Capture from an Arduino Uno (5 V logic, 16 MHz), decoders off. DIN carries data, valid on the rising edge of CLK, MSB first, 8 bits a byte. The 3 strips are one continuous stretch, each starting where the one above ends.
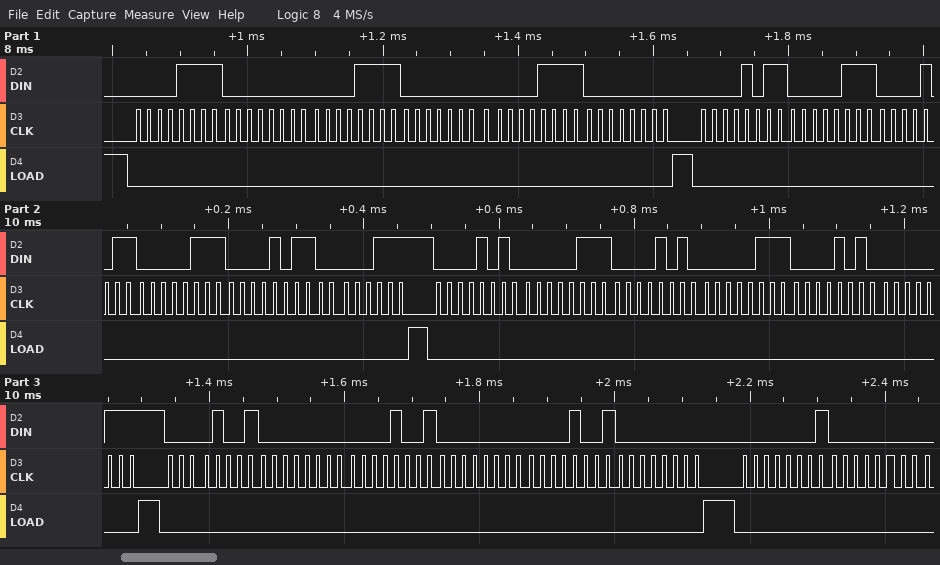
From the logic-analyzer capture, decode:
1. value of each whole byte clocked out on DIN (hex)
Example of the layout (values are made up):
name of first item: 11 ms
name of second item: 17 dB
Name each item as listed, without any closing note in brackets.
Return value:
value of each whole byte clocked out on DIN: 0x0F 0x00 0x0F 0x00 0x0F 0x00 0x0B 0x07 0x0B 0x07 0x0B 0x07 0x0A 0x07 0x0A 0x07 0x0A 0x07 0x09 0x00 0x09 0x00 0x09 0x00 0x01 0x00
